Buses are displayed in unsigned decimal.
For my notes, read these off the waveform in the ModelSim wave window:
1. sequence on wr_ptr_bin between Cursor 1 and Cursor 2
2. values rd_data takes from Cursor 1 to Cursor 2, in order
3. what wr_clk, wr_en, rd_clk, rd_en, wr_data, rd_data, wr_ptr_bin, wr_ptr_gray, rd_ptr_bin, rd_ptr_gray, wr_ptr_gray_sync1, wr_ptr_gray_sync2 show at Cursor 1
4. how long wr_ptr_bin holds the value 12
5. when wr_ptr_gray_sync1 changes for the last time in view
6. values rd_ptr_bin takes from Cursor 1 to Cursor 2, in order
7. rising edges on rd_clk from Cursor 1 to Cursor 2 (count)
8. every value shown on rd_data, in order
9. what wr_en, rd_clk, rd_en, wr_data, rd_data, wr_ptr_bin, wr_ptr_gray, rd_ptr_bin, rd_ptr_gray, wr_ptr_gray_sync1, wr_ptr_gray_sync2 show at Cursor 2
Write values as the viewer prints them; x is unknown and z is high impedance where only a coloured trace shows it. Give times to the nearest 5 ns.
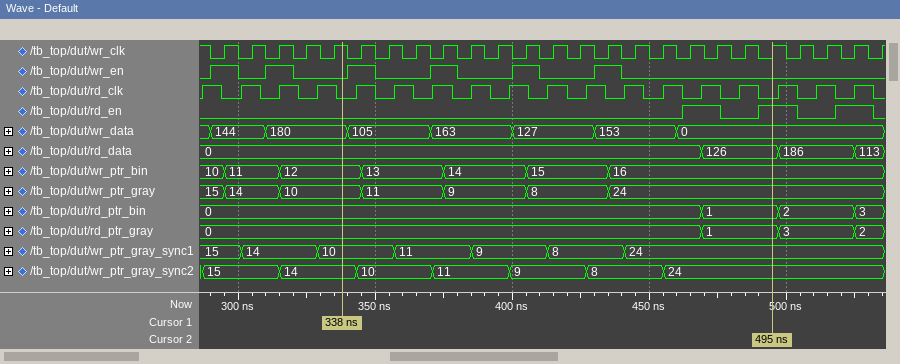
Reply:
12, 13, 14, 15, 16
0, 126
wr_clk=1, wr_en=0, rd_clk=0, rd_en=0, wr_data=180, rd_data=0, wr_ptr_bin=12, wr_ptr_gray=10, rd_ptr_bin=0, rd_ptr_gray=0, wr_ptr_gray_sync1=10, wr_ptr_gray_sync2=14
30 ns
440 ns
0, 1
11
0, 126, 186, 113
wr_en=0, rd_clk=0, rd_en=1, wr_data=0, rd_data=126, wr_ptr_bin=16, wr_ptr_gray=24, rd_ptr_bin=1, rd_ptr_gray=1, wr_ptr_gray_sync1=24, wr_ptr_gray_sync2=24
